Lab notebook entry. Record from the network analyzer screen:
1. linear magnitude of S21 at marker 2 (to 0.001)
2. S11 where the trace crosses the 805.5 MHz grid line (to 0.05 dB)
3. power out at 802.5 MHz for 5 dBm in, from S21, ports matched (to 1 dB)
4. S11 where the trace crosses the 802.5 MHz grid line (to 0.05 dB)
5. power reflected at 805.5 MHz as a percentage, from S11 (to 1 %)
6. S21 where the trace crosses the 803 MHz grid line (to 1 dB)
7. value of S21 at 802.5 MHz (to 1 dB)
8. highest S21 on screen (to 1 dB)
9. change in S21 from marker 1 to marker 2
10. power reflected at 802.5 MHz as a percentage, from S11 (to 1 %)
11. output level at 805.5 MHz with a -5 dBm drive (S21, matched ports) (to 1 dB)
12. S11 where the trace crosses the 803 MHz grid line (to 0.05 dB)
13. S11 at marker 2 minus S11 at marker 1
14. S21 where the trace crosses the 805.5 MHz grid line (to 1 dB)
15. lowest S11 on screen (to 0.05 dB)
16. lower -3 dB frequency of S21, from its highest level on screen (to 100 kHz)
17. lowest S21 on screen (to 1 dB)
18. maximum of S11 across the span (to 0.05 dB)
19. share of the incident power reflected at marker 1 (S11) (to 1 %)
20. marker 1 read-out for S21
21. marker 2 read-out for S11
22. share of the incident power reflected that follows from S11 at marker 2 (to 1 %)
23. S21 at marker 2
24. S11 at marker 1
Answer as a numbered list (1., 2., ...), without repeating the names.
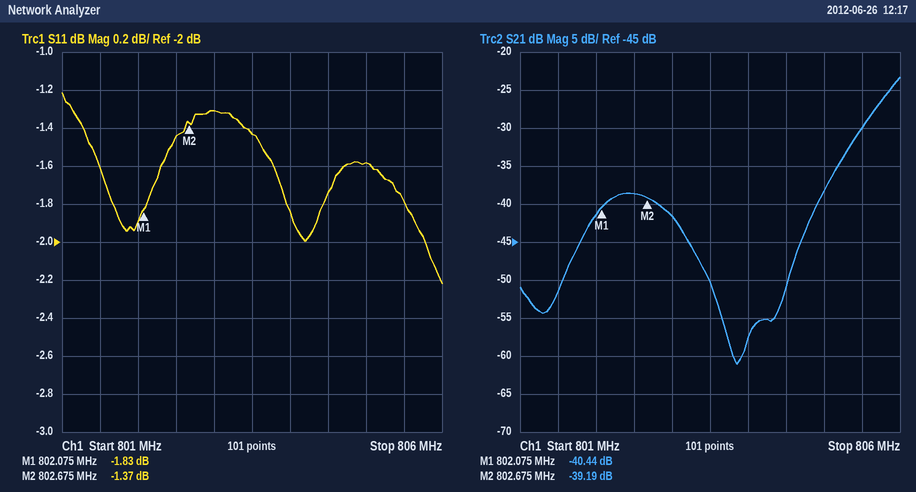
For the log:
1. 0.011
2. -1.80 dB
3. -34 dBm
4. -1.45 dB
5. 66 %
6. -42 dB
7. -39 dB
8. -23 dB
9. 1.25 dB
10. 72 %
11. -35 dBm
12. -1.30 dB
13. 0.46 dB
14. -30 dB
15. -2.20 dB
16. 805.8 MHz
17. -61 dB
18. -1.20 dB
19. 66 %
20. -40.44 dB
21. -1.37 dB
22. 73 %
23. -39.19 dB
24. -1.83 dB
